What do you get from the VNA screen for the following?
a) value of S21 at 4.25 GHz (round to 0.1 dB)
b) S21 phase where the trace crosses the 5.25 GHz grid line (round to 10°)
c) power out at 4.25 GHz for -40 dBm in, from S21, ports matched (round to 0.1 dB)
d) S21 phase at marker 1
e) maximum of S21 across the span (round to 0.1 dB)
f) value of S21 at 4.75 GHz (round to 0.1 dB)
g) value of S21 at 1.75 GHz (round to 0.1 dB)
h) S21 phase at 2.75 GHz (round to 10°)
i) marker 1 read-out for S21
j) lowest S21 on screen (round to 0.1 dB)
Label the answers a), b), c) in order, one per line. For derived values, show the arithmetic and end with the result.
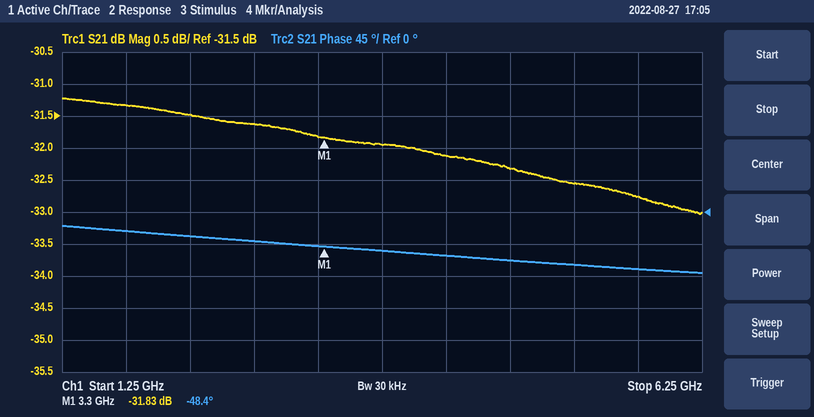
a) -32.1 dB
b) -70°
c) -40 dBm + (-32.1 dB) = -72.1 dBm
d) -48.4°
e) -31.2 dB
f) -32.3 dB
g) -31.3 dB
h) -40°
i) -31.83 dB
j) -33.0 dB
